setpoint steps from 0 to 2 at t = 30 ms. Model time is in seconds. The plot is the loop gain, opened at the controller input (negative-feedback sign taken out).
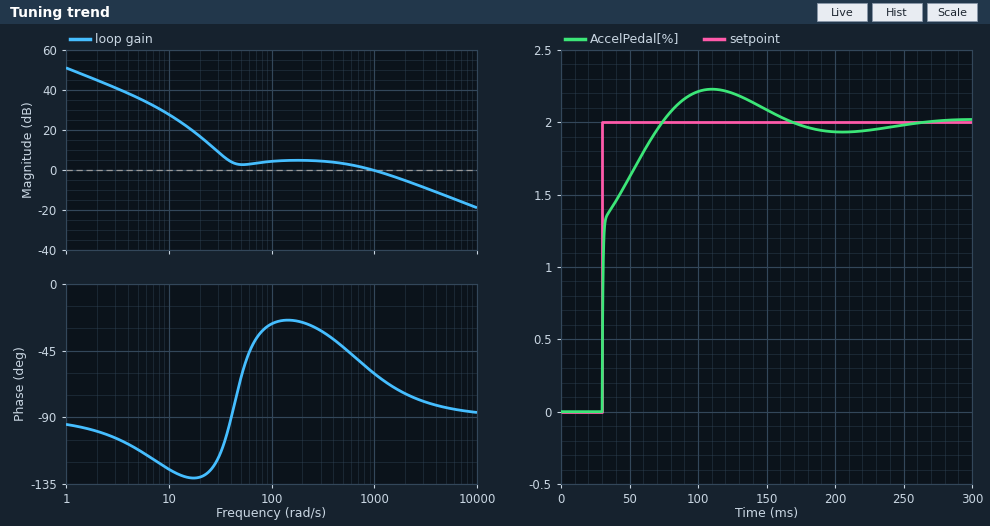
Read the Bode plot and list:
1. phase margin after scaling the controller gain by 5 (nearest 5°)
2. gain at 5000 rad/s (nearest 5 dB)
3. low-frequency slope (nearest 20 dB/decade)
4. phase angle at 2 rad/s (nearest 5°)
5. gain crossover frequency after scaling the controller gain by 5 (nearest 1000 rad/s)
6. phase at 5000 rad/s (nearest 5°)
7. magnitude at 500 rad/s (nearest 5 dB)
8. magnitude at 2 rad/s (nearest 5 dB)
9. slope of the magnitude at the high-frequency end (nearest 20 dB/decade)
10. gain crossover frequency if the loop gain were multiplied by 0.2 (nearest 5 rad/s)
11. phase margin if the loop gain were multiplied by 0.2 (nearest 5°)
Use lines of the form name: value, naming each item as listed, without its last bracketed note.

phase margin after scaling the controller gain by 5: 95°
gain at 5000 rad/s: -15 dB
low-frequency slope: -20 dB/decade
phase angle at 2 rad/s: -100°
gain crossover frequency after scaling the controller gain by 5: 6000 rad/s
phase at 5000 rad/s: -85°
magnitude at 500 rad/s: 5 dB
magnitude at 2 rad/s: 45 dB
slope of the magnitude at the high-frequency end: -20 dB/decade
gain crossover frequency if the loop gain were multiplied by 0.2: 25 rad/s
phase margin if the loop gain were multiplied by 0.2: 50°
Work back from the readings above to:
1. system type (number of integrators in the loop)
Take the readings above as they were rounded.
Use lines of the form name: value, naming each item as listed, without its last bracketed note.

system type: 1
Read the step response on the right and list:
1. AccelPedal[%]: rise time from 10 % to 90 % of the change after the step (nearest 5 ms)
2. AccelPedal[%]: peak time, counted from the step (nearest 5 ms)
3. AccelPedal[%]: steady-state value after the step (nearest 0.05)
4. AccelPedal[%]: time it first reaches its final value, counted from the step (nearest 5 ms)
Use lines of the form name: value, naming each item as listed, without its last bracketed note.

AccelPedal[%]: rise time from 10 % to 90 % of the change after the step: 30 ms
AccelPedal[%]: peak time, counted from the step: 80 ms
AccelPedal[%]: steady-state value after the step: 2.00
AccelPedal[%]: time it first reaches its final value, counted from the step: 45 ms
